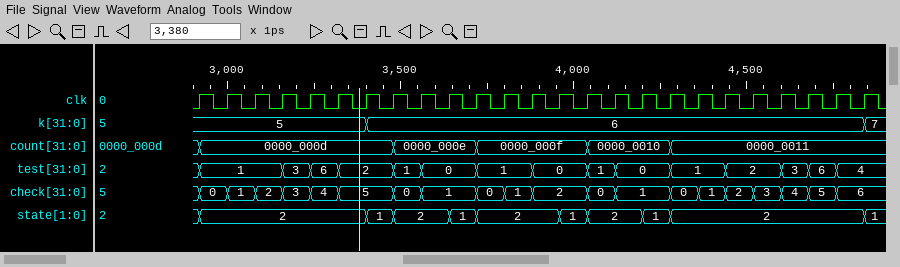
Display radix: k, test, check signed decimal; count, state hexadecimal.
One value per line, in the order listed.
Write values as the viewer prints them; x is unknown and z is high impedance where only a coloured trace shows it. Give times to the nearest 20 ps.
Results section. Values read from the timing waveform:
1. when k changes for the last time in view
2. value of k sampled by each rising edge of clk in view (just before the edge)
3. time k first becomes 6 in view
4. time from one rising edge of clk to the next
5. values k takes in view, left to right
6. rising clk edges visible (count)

4840 ps
5, 5, 5, 5, 5, 5, 5, 6, 6, 6, 6, 6, 6, 6, 6, 6, 6, 6, 6, 6, 6, 6, 6, 6, 6
3400 ps
80 ps
5, 6, 7
25
